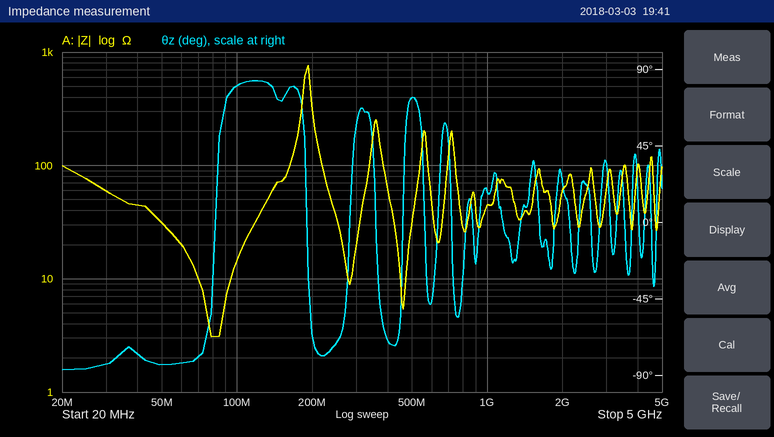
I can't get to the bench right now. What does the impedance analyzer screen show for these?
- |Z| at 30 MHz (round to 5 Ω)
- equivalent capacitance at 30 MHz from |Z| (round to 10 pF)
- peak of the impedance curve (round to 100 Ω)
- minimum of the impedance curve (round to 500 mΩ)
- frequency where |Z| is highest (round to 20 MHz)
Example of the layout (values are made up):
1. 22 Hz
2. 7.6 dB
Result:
1. 60 Ω
2. 90 pF
3. 800 Ω
4. 3.0 Ω
5. 200 MHz
